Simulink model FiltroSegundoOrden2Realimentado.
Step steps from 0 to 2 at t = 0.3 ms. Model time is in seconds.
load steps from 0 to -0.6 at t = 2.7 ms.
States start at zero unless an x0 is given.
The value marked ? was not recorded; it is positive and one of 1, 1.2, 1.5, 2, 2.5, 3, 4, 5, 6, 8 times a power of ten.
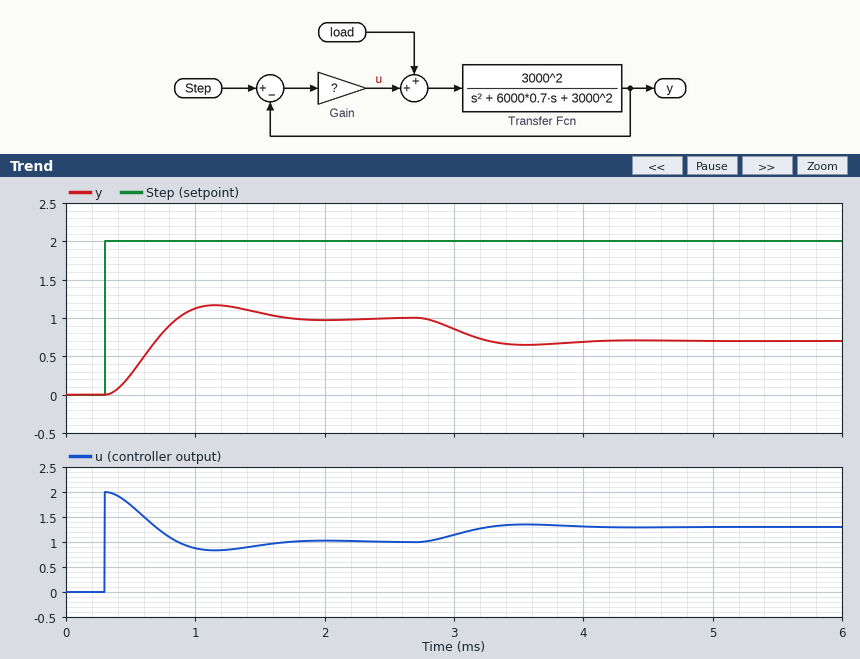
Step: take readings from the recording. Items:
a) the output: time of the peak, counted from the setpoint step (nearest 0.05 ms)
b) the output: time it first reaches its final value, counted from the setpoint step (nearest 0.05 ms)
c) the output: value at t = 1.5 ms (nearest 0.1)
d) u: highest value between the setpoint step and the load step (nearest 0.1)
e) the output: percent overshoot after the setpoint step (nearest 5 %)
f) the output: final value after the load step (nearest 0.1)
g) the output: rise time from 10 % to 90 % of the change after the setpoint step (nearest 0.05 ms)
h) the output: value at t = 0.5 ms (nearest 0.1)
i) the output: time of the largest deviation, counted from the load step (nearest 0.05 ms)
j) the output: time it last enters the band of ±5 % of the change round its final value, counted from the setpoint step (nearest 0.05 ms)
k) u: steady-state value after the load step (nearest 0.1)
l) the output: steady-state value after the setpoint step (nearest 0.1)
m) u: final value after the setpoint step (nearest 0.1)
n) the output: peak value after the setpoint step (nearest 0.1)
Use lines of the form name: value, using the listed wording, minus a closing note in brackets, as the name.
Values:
the output: time of the peak, counted from the setpoint step: 0.85 ms
the output: time it first reaches its final value, counted from the setpoint step: 0.55 ms
the output: value at t = 1.5 ms: 1.1
u: highest value between the setpoint step and the load step: 2.0
the output: percent overshoot after the setpoint step: 15 %
the output: final value after the load step: 0.7
the output: rise time from 10 % to 90 % of the change after the setpoint step: 0.40 ms
the output: value at t = 0.5 ms: 0.3
the output: time of the largest deviation, counted from the load step: 0.85 ms
the output: time it last enters the band of ±5 % of the change round its final value, counted from the setpoint step: 1.25 ms
u: steady-state value after the load step: 1.3
the output: steady-state value after the setpoint step: 1.0
u: final value after the setpoint step: 1.0
the output: peak value after the setpoint step: 1.2
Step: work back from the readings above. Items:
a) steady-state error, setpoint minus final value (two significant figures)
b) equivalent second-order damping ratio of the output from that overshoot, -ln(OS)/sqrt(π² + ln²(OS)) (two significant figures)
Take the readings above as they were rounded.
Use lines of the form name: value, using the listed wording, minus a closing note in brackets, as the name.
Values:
steady-state error, setpoint minus final value: 1.0
equivalent second-order damping ratio of the output from that overshoot, -ln(OS)/sqrt(π² + ln²(OS)): 0.52
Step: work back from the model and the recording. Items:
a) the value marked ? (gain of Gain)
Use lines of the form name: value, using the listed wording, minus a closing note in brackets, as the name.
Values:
the value marked ?: 1
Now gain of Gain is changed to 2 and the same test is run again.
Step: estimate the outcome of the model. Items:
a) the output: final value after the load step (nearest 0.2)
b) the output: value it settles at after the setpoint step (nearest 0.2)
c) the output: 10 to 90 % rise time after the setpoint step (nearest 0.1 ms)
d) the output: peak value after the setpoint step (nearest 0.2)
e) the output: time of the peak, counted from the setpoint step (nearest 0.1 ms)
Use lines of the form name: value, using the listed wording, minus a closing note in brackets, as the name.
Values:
the output: final value after the load step: 1.2
the output: value it settles at after the setpoint step: 1.4
the output: 10 to 90 % rise time after the setpoint step: 0.3 ms
the output: peak value after the setpoint step: 1.6
the output: time of the peak, counted from the setpoint step: 0.7 ms
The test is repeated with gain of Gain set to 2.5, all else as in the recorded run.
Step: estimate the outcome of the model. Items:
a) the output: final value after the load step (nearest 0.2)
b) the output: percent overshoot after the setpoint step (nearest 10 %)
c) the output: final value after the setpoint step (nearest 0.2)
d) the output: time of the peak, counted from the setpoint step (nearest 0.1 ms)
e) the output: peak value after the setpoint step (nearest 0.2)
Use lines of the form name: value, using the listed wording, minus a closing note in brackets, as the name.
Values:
the output: final value after the load step: 1.2
the output: percent overshoot after the setpoint step: 30 %
the output: final value after the setpoint step: 1.4
the output: time of the peak, counted from the setpoint step: 0.6 ms
the output: peak value after the setpoint step: 1.8
